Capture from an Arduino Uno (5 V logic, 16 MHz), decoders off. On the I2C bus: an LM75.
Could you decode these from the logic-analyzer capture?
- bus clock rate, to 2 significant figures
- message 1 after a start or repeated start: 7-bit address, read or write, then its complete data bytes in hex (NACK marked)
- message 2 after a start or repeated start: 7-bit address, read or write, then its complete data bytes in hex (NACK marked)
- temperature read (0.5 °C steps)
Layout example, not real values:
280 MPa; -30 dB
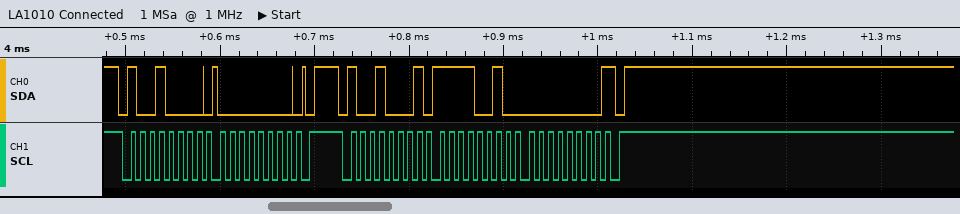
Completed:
100 kHz; 0x48 write: 00; 0x48 read: F2 00 NACK; -14.0 °C
